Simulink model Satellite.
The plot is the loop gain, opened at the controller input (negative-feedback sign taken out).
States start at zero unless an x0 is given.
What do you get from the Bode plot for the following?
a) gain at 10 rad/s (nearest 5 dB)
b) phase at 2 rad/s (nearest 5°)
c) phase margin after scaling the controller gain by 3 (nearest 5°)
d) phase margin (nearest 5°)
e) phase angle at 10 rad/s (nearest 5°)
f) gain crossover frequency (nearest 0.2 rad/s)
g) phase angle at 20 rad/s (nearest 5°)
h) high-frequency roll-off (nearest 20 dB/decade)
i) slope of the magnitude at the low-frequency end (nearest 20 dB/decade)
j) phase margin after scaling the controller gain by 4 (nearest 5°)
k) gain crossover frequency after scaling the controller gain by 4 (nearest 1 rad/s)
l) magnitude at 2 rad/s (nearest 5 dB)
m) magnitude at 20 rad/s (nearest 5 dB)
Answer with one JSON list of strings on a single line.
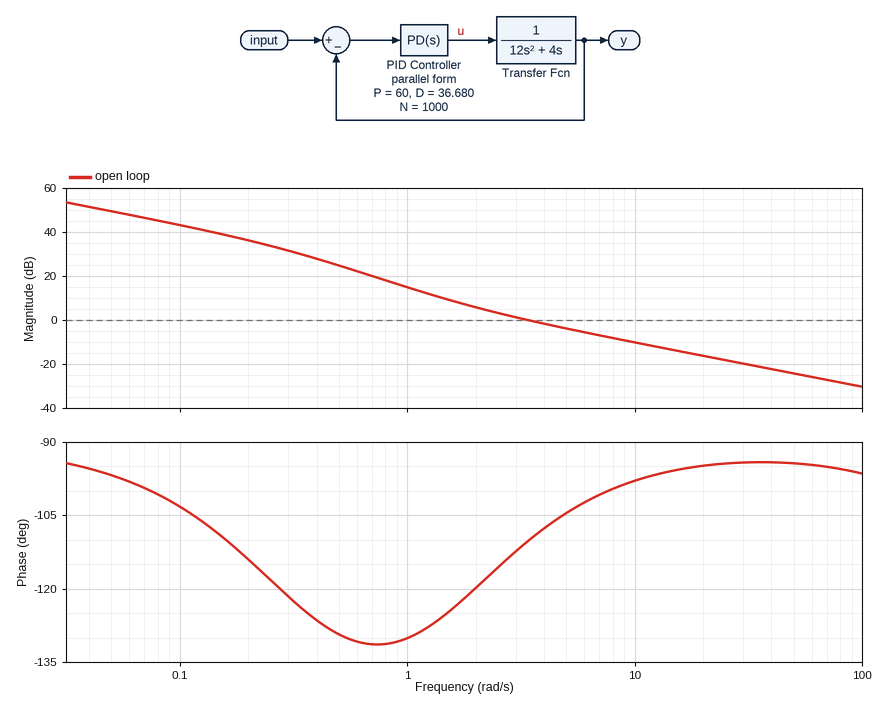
["-10 dB", "-120°", "80°", "70°", "-100°", "3.4 rad/s", "-95°", "-20 dB/decade", "-20 dB/decade", "85°", "12 rad/s", "5 dB", "-15 dB"]
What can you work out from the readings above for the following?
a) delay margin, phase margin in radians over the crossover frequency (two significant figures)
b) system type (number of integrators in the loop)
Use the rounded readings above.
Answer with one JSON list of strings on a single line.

["0.36 s", "1"]
